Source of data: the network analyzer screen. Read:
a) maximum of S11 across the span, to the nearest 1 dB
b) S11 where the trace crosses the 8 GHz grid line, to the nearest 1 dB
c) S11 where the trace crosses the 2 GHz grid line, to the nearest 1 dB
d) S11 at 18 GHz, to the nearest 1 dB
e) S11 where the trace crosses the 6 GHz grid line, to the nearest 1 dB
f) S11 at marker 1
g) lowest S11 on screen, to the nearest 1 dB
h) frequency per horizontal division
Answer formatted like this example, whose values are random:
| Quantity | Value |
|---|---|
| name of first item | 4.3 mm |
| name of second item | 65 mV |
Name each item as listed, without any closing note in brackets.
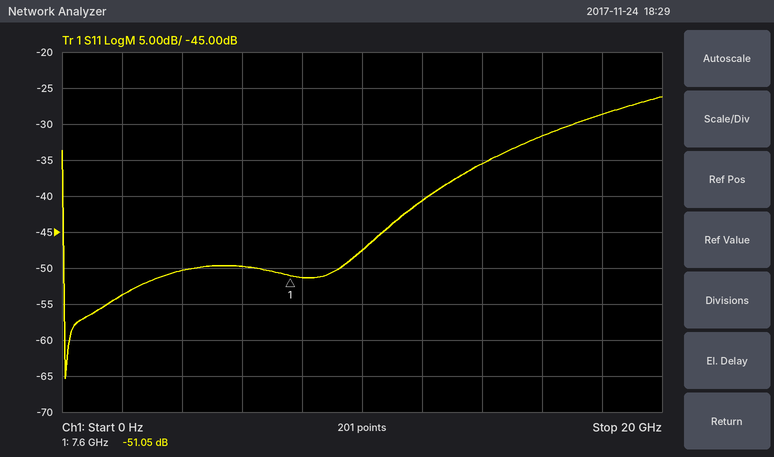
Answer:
| Quantity | Value |
|---|---|
| maximum of S11 across the span, to the nearest 1 dB | -26 dB |
| S11 where the trace crosses the 8 GHz grid line, to the nearest 1 dB | -51 dB |
| S11 where the trace crosses the 2 GHz grid line, to the nearest 1 dB | -54 dB |
| S11 at 18 GHz, to the nearest 1 dB | -29 dB |
| S11 where the trace crosses the 6 GHz grid line, to the nearest 1 dB | -50 dB |
| S11 at marker 1 | -51.05 dB |
| lowest S11 on screen, to the nearest 1 dB | -65 dB |
| frequency per horizontal division | 2 GHz |
